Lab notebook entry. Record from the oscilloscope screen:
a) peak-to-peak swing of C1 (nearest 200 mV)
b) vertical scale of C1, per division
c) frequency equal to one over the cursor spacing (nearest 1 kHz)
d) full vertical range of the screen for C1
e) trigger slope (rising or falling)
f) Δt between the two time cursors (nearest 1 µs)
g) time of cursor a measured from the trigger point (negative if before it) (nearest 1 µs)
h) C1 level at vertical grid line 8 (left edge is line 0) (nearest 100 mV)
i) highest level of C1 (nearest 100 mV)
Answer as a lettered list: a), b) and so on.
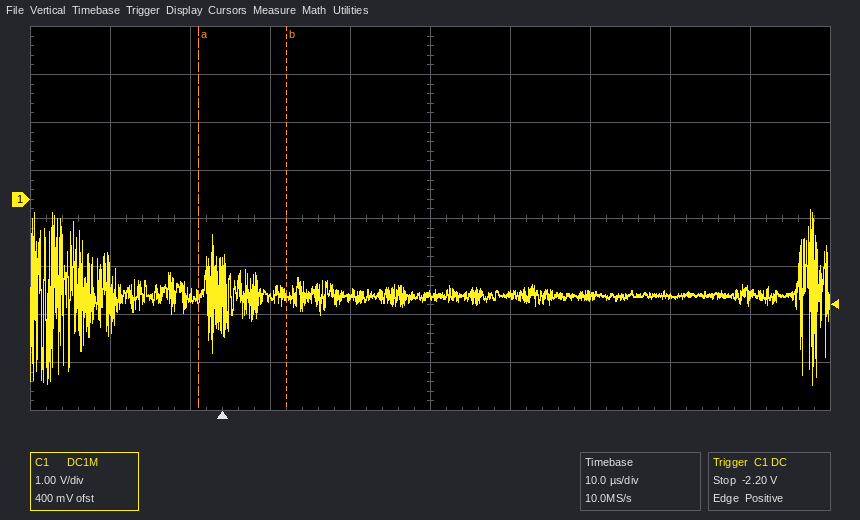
a) 3.6 V
b) 1 V
c) 91 kHz
d) 8 V
e) rising
f) 11 µs
g) -3 µs
h) -2.0 V
i) -200 mV
